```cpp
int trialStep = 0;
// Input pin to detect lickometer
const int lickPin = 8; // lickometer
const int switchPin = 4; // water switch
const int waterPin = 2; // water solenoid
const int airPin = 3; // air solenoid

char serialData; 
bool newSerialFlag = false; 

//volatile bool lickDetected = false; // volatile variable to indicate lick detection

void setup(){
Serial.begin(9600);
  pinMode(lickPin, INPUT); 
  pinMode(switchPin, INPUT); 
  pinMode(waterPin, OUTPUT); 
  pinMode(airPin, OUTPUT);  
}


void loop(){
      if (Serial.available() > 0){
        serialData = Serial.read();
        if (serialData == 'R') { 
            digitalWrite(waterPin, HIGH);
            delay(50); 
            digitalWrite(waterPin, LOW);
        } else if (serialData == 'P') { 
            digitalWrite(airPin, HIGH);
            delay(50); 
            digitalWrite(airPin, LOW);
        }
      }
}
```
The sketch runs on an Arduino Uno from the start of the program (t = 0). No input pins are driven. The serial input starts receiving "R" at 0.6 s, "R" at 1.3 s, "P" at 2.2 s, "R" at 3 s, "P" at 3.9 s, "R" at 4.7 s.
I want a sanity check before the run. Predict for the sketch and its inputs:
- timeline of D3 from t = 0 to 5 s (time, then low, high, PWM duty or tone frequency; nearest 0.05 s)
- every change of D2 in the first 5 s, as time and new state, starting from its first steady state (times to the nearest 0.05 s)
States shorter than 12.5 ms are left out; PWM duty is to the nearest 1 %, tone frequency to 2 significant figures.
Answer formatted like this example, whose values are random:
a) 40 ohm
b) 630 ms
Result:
a) 0 s low; 2.2 s high; 2.25 s low; 3.9 s high; 3.95 s low
b) 0 s low; 0.6 s high; 0.65 s low; 1.3 s high; 1.35 s low; 3 s high; 3.05 s low; 4.7 s high; 4.75 s low
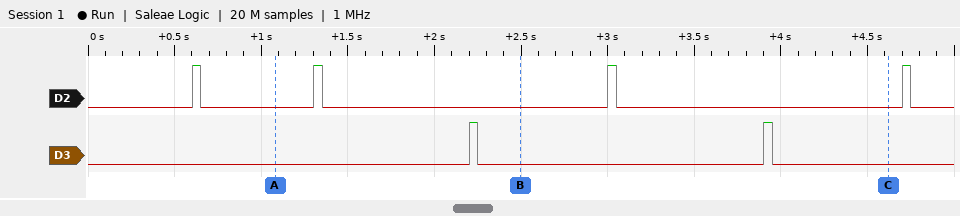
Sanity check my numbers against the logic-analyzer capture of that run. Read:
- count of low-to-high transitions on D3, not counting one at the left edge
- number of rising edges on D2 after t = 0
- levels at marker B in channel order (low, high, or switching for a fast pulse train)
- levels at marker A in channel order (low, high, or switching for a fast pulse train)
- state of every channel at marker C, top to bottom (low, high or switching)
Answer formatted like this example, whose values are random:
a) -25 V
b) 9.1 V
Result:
a) 2
b) 4
c) D2 low, D3 low
d) D2 low, D3 low
e) D2 low, D3 low
